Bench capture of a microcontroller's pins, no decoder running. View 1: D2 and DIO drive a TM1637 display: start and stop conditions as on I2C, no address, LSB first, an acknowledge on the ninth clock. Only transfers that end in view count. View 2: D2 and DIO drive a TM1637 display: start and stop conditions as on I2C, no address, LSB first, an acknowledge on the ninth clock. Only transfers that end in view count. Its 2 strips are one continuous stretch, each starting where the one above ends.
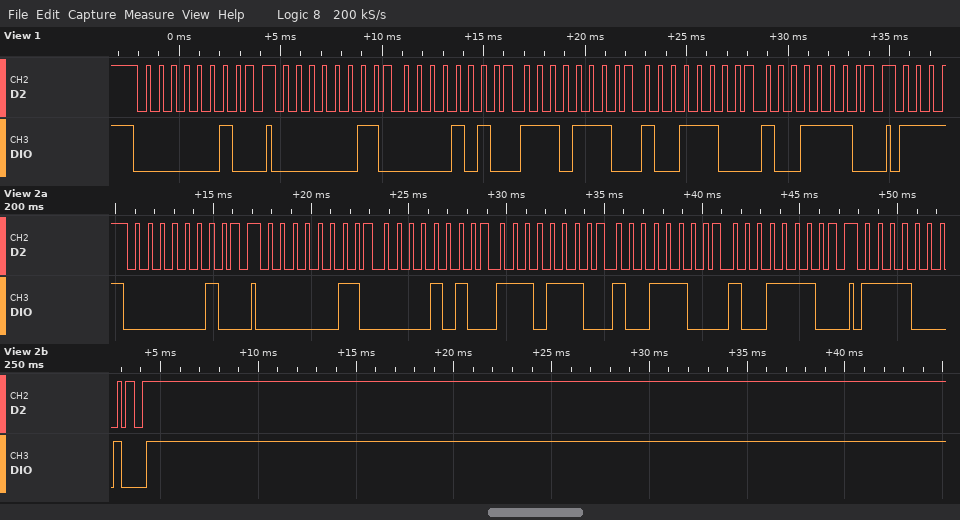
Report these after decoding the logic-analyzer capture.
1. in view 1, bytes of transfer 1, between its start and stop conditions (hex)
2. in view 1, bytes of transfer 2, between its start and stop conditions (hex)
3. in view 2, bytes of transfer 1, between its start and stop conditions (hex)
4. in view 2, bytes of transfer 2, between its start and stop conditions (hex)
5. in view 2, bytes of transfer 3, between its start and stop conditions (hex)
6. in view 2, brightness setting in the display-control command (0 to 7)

40
C0 50 77 39 79
40
C0 50 77 39 79
8F
7
